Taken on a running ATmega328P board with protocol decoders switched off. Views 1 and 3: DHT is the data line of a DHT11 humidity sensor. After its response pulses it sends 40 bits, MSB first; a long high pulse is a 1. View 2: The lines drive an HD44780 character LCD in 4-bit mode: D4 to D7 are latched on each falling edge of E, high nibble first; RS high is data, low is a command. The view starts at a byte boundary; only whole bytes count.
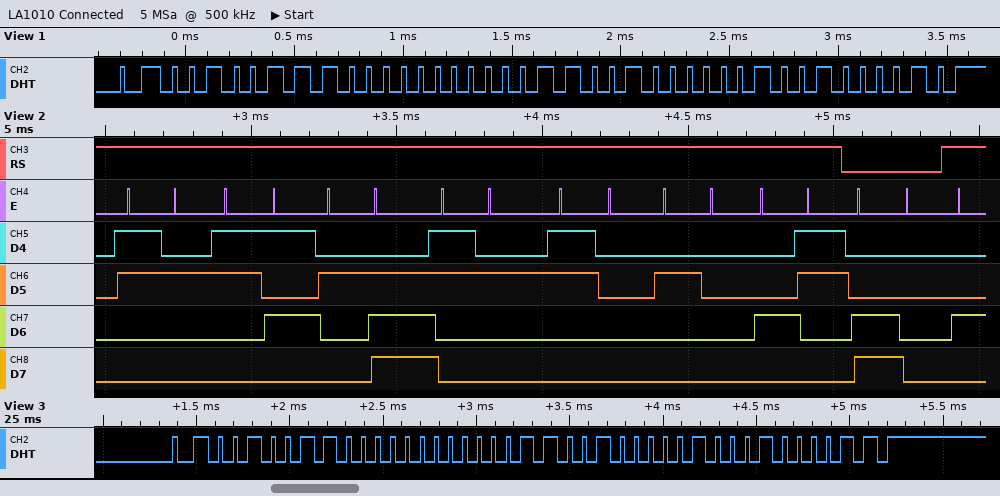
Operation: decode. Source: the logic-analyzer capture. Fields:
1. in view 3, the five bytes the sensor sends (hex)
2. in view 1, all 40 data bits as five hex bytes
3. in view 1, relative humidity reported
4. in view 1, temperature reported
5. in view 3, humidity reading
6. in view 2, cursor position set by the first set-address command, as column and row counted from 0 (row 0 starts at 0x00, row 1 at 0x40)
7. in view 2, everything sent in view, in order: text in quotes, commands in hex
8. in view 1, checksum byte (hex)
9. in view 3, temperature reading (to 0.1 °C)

26 00 19 04 43
27 00 19 02 42
39 %
25.2 °C
38 %
column 0, row 1
"25.20 C" 0xC0
0x42
25.4 °C
